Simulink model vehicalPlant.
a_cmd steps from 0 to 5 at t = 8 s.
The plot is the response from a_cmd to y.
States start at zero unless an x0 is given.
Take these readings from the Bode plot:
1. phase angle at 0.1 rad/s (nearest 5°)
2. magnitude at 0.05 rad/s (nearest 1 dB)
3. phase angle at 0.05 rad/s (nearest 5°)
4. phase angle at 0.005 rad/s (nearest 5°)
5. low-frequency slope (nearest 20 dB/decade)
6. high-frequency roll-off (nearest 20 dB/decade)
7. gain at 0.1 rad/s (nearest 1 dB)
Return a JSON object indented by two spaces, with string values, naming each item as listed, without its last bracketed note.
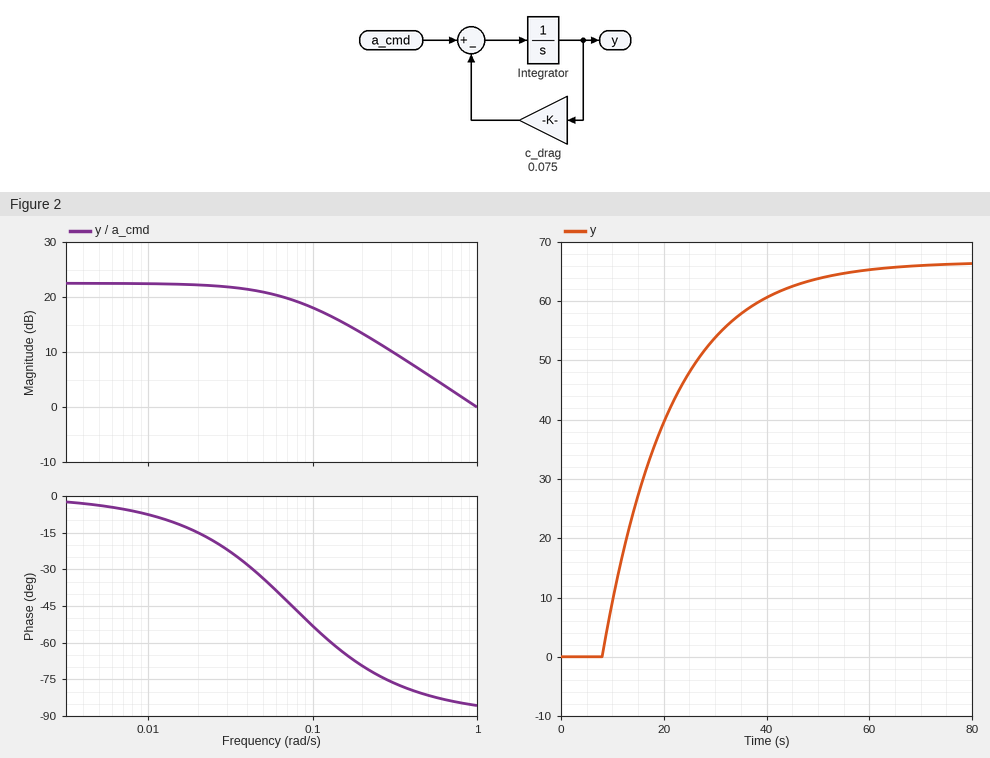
{
  "phase angle at 0.1 rad/s": "-55°",
  "magnitude at 0.05 rad/s": "21 dB",
  "phase angle at 0.05 rad/s": "-35°",
  "phase angle at 0.005 rad/s": "-5°",
  "low-frequency slope": "0 dB/decade",
  "high-frequency roll-off": "-20 dB/decade",
  "gain at 0.1 rad/s": "18 dB"
}
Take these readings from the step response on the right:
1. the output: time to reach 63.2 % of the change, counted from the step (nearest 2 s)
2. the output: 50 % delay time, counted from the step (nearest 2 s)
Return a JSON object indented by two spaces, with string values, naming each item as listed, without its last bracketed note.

{
  "the output: time to reach 63.2 % of the change, counted from the step": "14 s",
  "the output: 50 % delay time, counted from the step": "10 s"
}
